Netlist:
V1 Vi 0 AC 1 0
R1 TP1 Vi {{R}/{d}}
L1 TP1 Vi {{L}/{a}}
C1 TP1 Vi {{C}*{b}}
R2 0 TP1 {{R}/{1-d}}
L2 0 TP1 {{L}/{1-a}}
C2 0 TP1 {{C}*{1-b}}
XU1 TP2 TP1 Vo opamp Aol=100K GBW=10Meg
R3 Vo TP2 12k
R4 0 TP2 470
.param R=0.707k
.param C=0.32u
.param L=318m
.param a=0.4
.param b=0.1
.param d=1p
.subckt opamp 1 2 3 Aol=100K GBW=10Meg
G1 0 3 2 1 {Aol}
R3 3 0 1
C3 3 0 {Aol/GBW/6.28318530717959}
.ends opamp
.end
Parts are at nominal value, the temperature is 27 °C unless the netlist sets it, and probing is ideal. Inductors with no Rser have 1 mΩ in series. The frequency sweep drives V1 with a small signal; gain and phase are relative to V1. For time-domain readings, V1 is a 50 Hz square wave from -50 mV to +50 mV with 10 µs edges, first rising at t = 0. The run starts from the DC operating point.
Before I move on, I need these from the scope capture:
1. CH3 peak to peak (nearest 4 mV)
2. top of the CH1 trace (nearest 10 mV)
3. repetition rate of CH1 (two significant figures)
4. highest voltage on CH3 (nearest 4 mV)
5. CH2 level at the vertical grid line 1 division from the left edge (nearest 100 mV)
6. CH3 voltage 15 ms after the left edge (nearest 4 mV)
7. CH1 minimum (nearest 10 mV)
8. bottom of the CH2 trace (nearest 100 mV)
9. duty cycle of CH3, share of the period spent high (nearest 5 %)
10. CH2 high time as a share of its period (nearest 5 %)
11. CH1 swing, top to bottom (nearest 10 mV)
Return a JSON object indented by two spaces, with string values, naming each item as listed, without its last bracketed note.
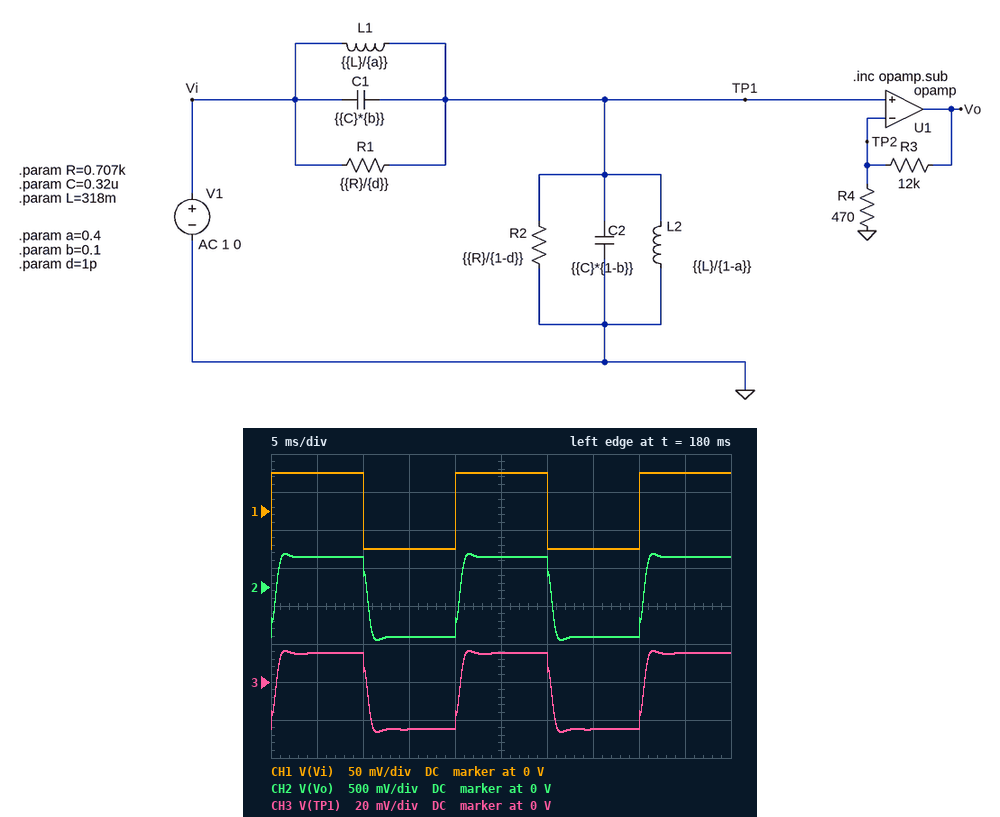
{
  "CH3 peak to peak": "44 mV",
  "top of the CH1 trace": "50 mV",
  "repetition rate of CH1": "50 Hz",
  "highest voltage on CH3": "16 mV",
  "CH2 level at the vertical grid line 1 division from the left edge": "400 mV",
  "CH3 voltage 15 ms after the left edge": "-24 mV",
  "CH1 minimum": "-50 mV",
  "bottom of the CH2 trace": "-700 mV",
  "duty cycle of CH3, share of the period spent high": "50 %",
  "CH2 high time as a share of its period": "50 %",
  "CH1 swing, top to bottom": "100 mV"
}
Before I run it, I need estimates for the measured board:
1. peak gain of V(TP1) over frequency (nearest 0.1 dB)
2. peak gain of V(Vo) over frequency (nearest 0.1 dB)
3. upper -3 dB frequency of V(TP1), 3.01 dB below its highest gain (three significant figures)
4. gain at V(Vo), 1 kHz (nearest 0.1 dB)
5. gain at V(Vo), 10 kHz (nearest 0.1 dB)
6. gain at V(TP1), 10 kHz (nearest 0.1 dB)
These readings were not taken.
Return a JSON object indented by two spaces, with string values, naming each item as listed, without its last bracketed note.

{
  "peak gain of V(TP1) over frequency": "-8.0 dB",
  "peak gain of V(Vo) over frequency": "20.5 dB",
  "upper -3 dB frequency of V(TP1), 3.01 dB below its highest gain": "400 Hz",
  "gain at V(Vo), 1 kHz": "-39.1 dB",
  "gain at V(Vo), 10 kHz": "8.4 dB",
  "gain at V(TP1), 10 kHz": "-20.1 dB"
}
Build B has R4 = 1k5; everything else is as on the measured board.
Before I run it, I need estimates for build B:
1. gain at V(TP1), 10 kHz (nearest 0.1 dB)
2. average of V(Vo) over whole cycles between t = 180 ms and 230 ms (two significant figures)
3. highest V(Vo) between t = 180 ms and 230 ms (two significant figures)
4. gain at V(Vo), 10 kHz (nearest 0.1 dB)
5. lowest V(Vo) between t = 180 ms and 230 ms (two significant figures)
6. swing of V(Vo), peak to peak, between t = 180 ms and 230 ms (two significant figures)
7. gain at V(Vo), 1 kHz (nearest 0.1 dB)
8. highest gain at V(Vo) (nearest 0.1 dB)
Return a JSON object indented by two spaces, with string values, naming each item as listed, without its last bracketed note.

{
  "gain at V(TP1), 10 kHz": "-20.1 dB",
  "average of V(Vo) over whole cycles between t = 180 ms and 230 ms": "-45 mV",
  "highest V(Vo) between t = 180 ms and 230 ms": "150 mV",
  "gain at V(Vo), 10 kHz": "-1.0 dB",
  "lowest V(Vo) between t = 180 ms and 230 ms": "-240 mV",
  "swing of V(Vo), peak to peak, between t = 180 ms and 230 ms": "390 mV",
  "gain at V(Vo), 1 kHz": "-48.5 dB",
  "highest gain at V(Vo)": "11.1 dB"
}
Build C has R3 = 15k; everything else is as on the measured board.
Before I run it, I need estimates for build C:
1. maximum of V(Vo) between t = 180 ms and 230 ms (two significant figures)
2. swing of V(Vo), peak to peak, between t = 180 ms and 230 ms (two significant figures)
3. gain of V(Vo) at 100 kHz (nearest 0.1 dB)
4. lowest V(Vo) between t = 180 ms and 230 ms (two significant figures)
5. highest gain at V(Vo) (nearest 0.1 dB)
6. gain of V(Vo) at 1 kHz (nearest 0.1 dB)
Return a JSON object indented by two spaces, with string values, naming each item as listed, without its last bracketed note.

{
  "maximum of V(Vo) between t = 180 ms and 230 ms": "540 mV",
  "swing of V(Vo), peak to peak, between t = 180 ms and 230 ms": "1.4 V",
  "gain of V(Vo) at 100 kHz": "9.9 dB",
  "lowest V(Vo) between t = 180 ms and 230 ms": "-870 mV",
  "highest gain at V(Vo)": "22.4 dB",
  "gain of V(Vo) at 1 kHz": "-37.2 dB"
}
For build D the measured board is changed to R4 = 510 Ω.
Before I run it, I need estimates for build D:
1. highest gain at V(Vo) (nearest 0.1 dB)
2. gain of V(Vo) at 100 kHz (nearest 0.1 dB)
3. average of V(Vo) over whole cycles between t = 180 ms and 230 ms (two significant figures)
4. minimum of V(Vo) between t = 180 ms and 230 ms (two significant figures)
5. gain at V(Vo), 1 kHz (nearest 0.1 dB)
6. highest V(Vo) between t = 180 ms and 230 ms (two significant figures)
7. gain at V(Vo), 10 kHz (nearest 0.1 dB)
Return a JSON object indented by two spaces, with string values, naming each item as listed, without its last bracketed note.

{
  "highest gain at V(Vo)": "19.8 dB",
  "gain of V(Vo) at 100 kHz": "7.5 dB",
  "average of V(Vo) over whole cycles between t = 180 ms and 230 ms": "-120 mV",
  "minimum of V(Vo) between t = 180 ms and 230 ms": "-650 mV",
  "gain at V(Vo), 1 kHz": "-39.8 dB",
  "highest V(Vo) between t = 180 ms and 230 ms": "400 mV",
  "gain at V(Vo), 10 kHz": "7.7 dB"
}
